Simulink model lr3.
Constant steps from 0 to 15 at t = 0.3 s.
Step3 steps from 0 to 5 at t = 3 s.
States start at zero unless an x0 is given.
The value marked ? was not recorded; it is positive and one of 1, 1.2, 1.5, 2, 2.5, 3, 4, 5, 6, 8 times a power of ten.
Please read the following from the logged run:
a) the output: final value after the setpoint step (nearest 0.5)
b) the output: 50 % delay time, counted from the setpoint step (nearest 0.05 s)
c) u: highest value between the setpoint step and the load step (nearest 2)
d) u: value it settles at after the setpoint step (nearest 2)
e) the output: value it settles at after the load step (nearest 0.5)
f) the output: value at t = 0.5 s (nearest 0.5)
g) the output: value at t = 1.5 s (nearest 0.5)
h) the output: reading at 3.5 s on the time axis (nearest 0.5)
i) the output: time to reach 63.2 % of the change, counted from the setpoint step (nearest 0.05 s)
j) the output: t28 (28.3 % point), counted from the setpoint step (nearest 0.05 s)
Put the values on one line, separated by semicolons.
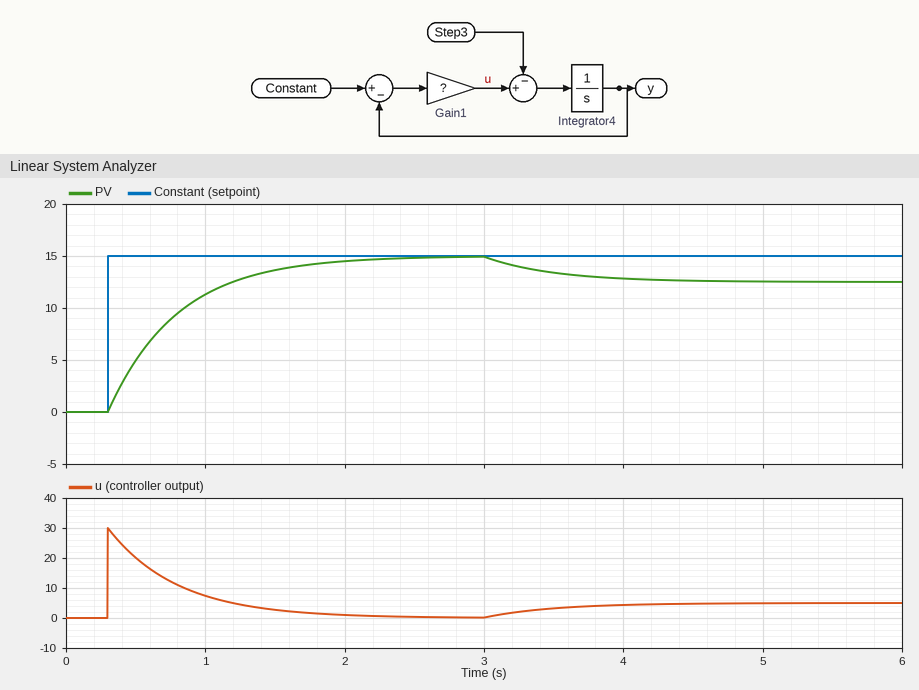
15.0; 0.35 s; 30; 0; 12.5; 5.0; 13.5; 13.5; 0.50 s; 0.15 s
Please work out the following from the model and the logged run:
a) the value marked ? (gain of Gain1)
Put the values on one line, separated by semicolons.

2
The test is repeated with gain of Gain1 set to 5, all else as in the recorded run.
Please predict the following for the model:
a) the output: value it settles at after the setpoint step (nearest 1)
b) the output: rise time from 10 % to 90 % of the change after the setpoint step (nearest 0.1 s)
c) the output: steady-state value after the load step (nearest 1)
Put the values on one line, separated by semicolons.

15; 0.4 s; 14
